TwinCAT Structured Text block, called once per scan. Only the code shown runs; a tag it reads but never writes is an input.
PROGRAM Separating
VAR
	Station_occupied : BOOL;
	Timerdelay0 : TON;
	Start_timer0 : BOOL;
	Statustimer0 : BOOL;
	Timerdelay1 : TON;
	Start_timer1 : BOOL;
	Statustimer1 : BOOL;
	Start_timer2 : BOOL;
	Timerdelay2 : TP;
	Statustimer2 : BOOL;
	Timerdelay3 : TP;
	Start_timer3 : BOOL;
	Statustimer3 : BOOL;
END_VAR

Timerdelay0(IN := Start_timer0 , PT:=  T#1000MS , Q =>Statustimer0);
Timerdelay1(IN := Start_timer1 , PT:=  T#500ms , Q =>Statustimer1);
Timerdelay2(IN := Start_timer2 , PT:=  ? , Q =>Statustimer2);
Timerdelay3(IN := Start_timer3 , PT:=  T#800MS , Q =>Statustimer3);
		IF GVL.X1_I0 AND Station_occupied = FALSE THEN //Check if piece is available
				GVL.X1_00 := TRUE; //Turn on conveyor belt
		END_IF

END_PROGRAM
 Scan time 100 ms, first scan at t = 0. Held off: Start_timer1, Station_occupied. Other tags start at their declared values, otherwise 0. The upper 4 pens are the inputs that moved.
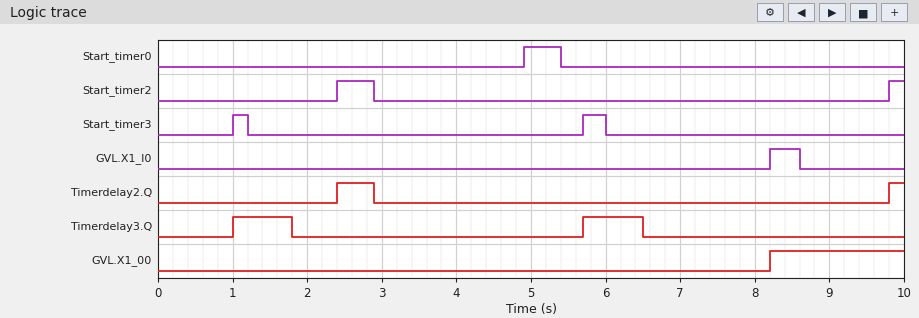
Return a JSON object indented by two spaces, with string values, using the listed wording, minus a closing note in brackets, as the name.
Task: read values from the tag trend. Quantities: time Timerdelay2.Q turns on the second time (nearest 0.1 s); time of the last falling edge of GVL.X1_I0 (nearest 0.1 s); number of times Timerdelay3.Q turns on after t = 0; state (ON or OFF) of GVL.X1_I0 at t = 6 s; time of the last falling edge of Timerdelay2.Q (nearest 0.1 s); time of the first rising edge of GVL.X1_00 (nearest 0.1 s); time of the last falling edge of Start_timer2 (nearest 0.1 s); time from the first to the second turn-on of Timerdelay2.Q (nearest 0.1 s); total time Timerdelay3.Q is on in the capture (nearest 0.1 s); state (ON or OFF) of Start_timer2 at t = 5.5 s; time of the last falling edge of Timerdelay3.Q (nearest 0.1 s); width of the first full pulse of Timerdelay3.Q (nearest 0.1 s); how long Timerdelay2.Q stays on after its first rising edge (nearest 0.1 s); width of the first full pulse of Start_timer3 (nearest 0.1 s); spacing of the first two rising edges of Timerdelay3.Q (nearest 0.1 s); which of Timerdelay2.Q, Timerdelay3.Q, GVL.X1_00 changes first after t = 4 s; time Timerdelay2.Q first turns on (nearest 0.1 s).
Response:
{
  "time Timerdelay2.Q turns on the second time": "9.8 s",
  "time of the last falling edge of GVL.X1_I0": "8.6 s",
  "number of times Timerdelay3.Q turns on after t = 0": "2",
  "state (ON or OFF) of GVL.X1_I0 at t = 6 s": "OFF",
  "time of the last falling edge of Timerdelay2.Q": "2.9 s",
  "time of the first rising edge of GVL.X1_00": "8.2 s",
  "time of the last falling edge of Start_timer2": "2.9 s",
  "time from the first to the second turn-on of Timerdelay2.Q": "7.4 s",
  "total time Timerdelay3.Q is on in the capture": "1.6 s",
  "state (ON or OFF) of Start_timer2 at t = 5.5 s": "OFF",
  "time of the last falling edge of Timerdelay3.Q": "6.5 s",
  "width of the first full pulse of Timerdelay3.Q": "0.8 s",
  "how long Timerdelay2.Q stays on after its first rising edge": "0.5 s",
  "width of the first full pulse of Start_timer3": "0.2 s",
  "spacing of the first two rising edges of Timerdelay3.Q": "4.7 s",
  "which of Timerdelay2.Q, Timerdelay3.Q, GVL.X1_00 changes first after t = 4 s": "Timerdelay3.Q",
  "time Timerdelay2.Q first turns on": "2.4 s"
}
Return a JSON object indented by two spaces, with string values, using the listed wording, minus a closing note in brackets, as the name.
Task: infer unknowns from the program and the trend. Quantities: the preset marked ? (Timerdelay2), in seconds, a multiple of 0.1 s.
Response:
{
  "the preset marked ? (Timerdelay2), in seconds, a multiple of 0.1 s": "0.5 s"
}
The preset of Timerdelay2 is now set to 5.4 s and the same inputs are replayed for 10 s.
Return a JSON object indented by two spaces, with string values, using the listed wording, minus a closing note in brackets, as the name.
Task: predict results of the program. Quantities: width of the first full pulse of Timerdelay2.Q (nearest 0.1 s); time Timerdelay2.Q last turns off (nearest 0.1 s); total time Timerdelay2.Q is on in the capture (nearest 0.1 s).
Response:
{
  "width of the first full pulse of Timerdelay2.Q": "5.4 s",
  "time Timerdelay2.Q last turns off": "7.8 s",
  "total time Timerdelay2.Q is on in the capture": "5.6 s"
}
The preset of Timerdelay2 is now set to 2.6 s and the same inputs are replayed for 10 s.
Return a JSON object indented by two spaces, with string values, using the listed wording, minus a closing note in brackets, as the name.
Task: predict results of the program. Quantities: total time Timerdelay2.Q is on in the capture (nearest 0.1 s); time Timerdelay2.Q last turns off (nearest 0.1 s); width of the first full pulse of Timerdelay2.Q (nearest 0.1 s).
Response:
{
  "total time Timerdelay2.Q is on in the capture": "2.8 s",
  "time Timerdelay2.Q last turns off": "5.0 s",
  "width of the first full pulse of Timerdelay2.Q": "2.6 s"
}
